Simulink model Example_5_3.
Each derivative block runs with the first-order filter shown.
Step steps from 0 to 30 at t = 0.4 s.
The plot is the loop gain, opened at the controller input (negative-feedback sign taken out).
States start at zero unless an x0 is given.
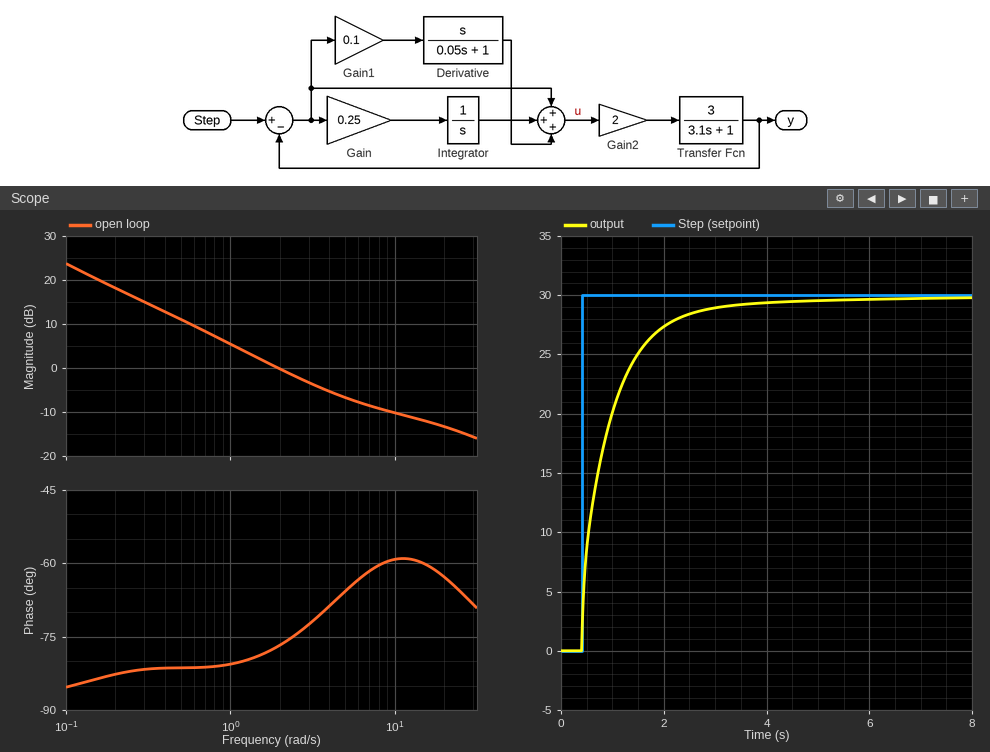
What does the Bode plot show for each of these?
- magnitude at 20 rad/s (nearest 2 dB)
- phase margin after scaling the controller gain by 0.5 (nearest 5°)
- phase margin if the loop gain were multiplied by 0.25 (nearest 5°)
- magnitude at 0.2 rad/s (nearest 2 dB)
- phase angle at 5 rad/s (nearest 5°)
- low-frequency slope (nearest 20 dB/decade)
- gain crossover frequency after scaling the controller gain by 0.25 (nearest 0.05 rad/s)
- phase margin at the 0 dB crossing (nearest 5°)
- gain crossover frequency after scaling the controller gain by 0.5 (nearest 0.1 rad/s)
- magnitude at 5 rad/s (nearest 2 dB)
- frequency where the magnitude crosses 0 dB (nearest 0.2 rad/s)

-14 dB
100°
100°
18 dB
-65°
-20 dB/decade
0.45 rad/s
105°
0.9 rad/s
-6 dB
2.0 rad/s
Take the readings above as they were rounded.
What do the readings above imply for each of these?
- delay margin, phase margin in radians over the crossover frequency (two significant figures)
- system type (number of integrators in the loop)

0.92 s
1
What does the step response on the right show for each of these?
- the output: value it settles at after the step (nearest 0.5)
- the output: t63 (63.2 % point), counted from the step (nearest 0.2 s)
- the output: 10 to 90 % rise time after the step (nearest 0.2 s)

30.0
0.6 s
1.4 s
